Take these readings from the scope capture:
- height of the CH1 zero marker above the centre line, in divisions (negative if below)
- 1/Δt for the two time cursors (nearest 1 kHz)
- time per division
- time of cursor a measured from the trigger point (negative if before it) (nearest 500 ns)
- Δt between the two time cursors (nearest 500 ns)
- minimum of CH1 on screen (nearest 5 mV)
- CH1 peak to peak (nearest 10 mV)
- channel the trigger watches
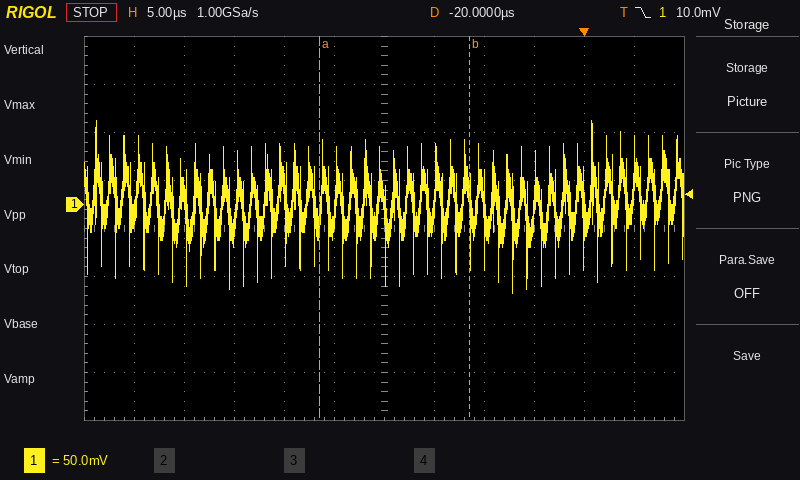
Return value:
+0.5 div
67 kHz
5 µs
-26.5 µs
15.0 µs
-90 mV
180 mV
CH1
